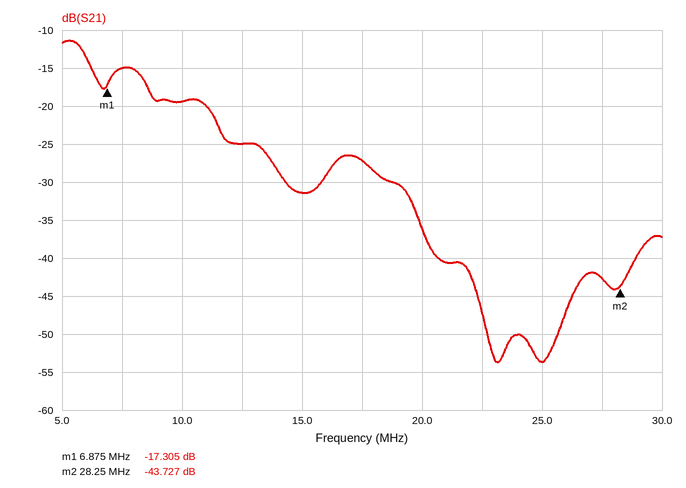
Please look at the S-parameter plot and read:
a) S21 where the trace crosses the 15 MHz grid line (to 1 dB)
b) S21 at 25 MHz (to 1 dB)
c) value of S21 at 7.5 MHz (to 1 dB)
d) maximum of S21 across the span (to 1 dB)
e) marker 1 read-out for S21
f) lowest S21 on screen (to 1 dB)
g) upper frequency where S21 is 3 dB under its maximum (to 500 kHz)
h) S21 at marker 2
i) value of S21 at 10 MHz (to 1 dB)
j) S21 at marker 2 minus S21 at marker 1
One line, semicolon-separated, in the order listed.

-31 dB; -54 dB; -15 dB; -11 dB; -17.305 dB; -54 dB; 6.0 MHz; -43.727 dB; -19 dB; -26.422 dB
